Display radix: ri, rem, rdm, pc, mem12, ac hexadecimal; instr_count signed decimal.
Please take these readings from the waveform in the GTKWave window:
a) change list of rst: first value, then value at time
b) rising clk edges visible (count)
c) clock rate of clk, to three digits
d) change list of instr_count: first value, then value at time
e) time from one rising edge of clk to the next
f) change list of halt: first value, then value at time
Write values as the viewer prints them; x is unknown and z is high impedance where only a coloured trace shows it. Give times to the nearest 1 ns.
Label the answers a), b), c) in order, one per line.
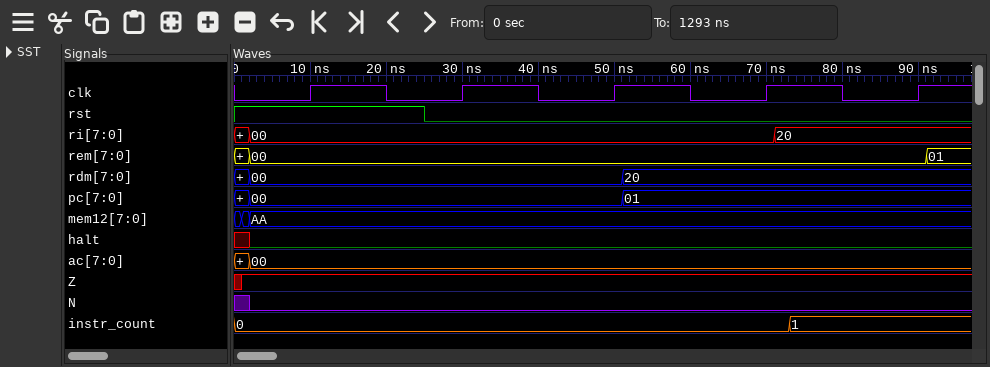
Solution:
a) 1, 0 at 25 ns
b) 5
c) 50.0 MHz
d) 0, 1 at 73 ns
e) 20 ns
f) x, 0 at 2 ns
